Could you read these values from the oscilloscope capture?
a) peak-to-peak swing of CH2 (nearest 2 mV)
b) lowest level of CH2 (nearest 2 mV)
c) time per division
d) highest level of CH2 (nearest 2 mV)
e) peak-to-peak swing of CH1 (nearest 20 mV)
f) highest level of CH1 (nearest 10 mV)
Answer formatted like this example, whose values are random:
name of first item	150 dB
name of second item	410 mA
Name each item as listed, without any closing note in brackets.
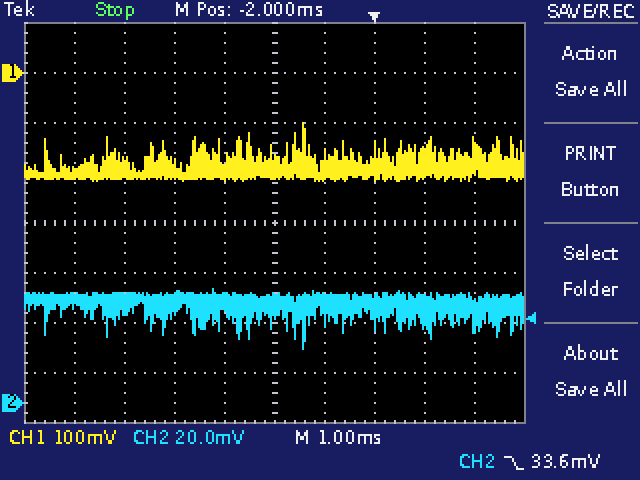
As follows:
peak-to-peak swing of CH2	24 mV
lowest level of CH2	22 mV
time per division	1 ms
highest level of CH2	46 mV
peak-to-peak swing of CH1	120 mV
highest level of CH1	-100 mV
